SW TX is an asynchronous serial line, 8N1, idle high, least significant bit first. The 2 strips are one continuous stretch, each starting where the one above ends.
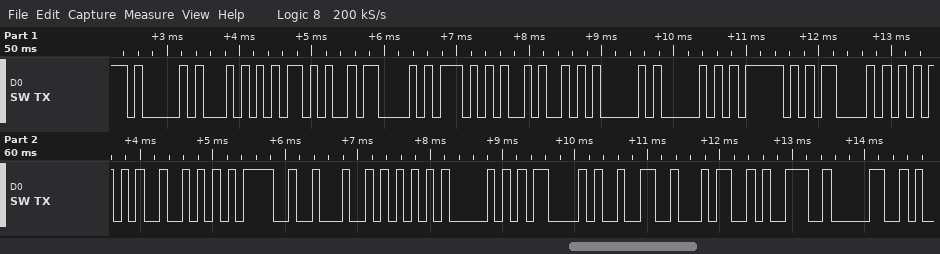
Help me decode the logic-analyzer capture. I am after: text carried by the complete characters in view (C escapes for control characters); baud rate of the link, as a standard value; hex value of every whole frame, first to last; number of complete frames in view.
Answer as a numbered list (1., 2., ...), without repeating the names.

1. "AT+CWJAP_CUR=\"UPC2490"
2. 9600 baud
3. 0x41 0x54 0x2B 0x43 0x57 0x4A 0x41 0x50 0x5F 0x43 0x55 0x52 0x3D 0x22 0x55 0x50 0x43 0x32 0x34 0x39 0x30
4. 21
